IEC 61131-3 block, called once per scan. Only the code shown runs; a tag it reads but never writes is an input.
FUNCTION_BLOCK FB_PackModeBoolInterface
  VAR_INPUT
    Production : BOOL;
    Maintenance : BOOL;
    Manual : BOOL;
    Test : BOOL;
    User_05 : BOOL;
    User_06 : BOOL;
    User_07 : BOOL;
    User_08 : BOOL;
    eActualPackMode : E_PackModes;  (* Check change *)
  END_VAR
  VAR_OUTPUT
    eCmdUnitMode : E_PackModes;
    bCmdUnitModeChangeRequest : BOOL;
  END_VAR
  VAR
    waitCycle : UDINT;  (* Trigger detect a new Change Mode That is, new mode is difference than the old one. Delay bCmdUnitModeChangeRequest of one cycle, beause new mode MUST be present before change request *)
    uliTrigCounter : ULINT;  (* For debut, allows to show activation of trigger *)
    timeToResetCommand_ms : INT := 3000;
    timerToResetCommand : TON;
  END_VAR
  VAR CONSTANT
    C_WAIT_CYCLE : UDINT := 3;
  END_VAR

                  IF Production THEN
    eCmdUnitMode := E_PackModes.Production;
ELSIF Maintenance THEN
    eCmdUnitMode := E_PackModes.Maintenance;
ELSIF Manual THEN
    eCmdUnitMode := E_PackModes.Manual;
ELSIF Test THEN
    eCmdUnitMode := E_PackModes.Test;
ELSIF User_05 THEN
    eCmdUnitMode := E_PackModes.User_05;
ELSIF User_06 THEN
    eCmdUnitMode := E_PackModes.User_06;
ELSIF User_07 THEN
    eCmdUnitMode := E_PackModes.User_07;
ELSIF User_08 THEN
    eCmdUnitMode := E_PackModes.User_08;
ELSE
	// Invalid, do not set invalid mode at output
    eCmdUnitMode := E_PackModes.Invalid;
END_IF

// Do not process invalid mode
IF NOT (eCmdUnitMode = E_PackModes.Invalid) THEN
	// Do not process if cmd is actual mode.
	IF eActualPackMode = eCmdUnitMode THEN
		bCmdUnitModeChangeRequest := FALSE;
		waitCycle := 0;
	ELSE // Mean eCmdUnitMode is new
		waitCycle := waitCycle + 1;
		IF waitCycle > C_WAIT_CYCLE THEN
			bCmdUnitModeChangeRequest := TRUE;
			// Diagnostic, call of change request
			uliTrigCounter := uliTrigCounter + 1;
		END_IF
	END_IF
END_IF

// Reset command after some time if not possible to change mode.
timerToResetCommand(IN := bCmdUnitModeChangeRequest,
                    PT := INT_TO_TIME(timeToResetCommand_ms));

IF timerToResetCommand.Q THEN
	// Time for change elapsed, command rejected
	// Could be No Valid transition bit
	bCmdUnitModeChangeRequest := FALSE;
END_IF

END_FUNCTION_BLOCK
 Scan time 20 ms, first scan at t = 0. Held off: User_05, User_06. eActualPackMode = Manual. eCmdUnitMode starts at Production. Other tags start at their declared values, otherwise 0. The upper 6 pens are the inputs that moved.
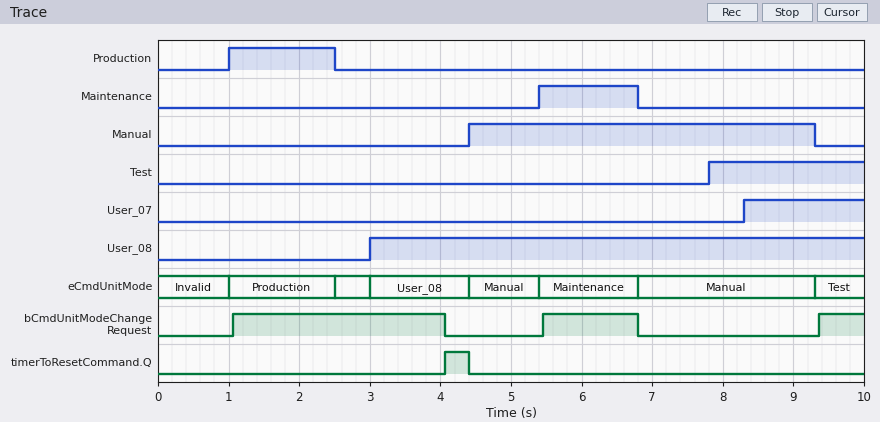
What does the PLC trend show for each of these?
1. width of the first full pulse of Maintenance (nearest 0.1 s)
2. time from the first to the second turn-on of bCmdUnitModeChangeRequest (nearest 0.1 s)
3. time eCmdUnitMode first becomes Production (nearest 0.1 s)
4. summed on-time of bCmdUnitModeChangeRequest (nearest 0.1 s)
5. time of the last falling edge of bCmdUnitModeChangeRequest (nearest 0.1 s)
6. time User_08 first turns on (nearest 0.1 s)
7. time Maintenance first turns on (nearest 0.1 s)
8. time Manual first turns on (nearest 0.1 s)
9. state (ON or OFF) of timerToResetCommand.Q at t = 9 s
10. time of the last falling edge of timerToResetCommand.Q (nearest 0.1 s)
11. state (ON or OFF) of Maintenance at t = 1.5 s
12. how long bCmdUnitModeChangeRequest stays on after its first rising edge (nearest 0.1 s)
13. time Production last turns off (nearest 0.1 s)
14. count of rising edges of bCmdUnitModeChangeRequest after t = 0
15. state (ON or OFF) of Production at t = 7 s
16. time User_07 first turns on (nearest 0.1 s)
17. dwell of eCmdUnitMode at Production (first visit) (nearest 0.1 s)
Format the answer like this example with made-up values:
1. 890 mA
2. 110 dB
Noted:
1. 1.4 s
2. 4.4 s
3. 1.0 s
4. 5.0 s
5. 6.8 s
6. 3.0 s
7. 5.4 s
8. 4.4 s
9. OFF
10. 4.4 s
11. OFF
12. 3.0 s
13. 2.5 s
14. 3
15. OFF
16. 8.3 s
17. 1.5 s
